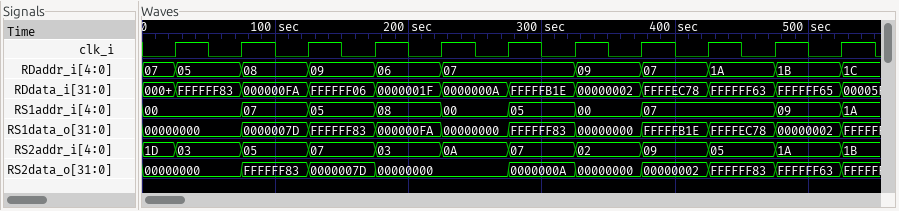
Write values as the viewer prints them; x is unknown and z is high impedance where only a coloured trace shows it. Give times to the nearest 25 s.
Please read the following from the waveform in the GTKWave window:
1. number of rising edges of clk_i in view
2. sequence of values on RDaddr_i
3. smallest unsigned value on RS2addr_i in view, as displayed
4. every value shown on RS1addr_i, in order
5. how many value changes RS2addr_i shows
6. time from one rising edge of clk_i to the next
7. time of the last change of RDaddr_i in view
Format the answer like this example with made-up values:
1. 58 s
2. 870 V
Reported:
1. 11
2. 07, 05, 08, 09, 06, 07, 09, 07, 1A, 1B, 1C
3. 02
4. 00, 07, 05, 08, 00, 05, 00, 07, 09, 1A
5. 11
6. 50 s
7. 525 s
